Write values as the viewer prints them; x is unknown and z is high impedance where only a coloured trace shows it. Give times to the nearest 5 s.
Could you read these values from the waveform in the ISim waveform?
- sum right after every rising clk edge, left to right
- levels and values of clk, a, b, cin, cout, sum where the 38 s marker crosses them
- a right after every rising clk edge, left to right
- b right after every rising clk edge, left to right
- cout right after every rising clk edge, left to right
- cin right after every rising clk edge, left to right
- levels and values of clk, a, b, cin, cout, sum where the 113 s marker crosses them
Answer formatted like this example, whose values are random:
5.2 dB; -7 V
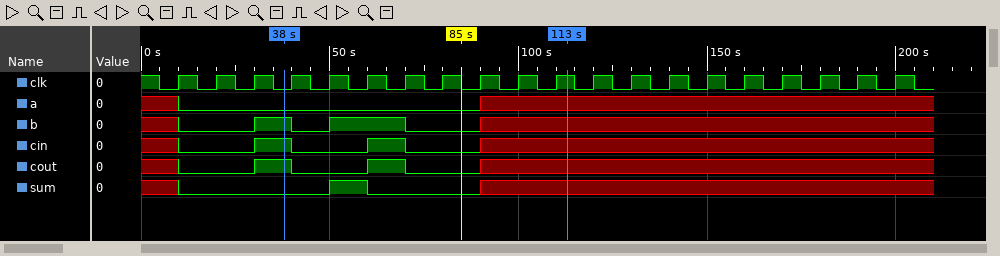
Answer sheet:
0 0 0 0 1 0 0 0 x x x x x x x x x x x x; clk=0, a=0, b=1, cin=1, cout=1, sum=0; 0 0 0 0 0 0 0 0 x x x x x x x x x x x x; 0 0 1 0 1 1 0 0 x x x x x x x x x x x x; 0 0 1 0 0 1 0 0 x x x x x x x x x x x x; 0 0 1 0 0 1 0 0 x x x x x x x x x x x x; clk=1, a=x, b=x, cin=x, cout=x, sum=x
